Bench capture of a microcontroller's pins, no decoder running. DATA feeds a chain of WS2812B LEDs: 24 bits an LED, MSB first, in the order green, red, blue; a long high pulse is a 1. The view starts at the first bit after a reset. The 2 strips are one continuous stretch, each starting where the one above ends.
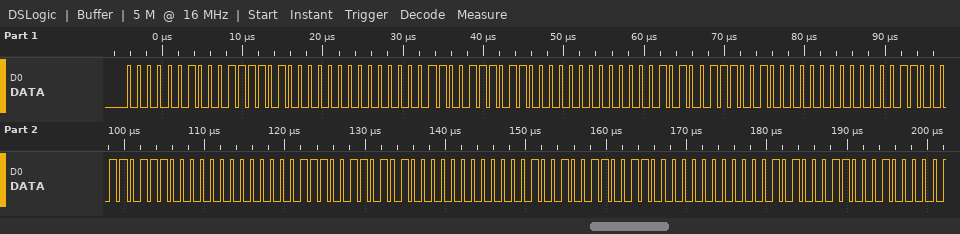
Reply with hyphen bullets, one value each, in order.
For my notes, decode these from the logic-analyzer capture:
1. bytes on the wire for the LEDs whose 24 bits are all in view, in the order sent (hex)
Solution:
- 02 3D 00 03 3B 00 05 39 00 06 37 00 07 35 00 09 33 00
